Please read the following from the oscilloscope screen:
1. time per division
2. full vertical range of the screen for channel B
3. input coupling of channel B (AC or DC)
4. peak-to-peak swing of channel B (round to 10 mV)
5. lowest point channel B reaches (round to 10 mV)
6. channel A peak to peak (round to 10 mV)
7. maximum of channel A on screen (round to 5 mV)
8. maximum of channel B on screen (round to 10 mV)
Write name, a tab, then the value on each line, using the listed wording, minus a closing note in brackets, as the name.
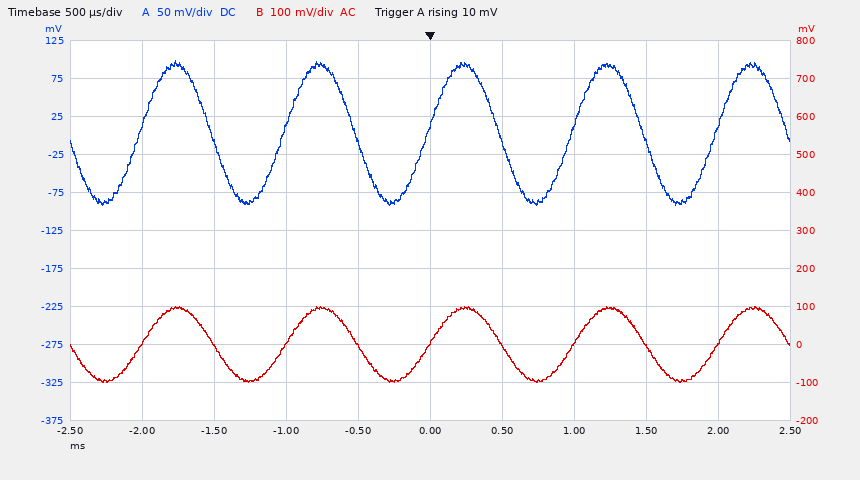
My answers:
time per division	500 µs
full vertical range of the screen for channel B	1 V
input coupling of channel B	AC
peak-to-peak swing of channel B	200 mV
lowest point channel B reaches	-100 mV
channel A peak to peak	190 mV
maximum of channel A on screen	100 mV
maximum of channel B on screen	100 mV
